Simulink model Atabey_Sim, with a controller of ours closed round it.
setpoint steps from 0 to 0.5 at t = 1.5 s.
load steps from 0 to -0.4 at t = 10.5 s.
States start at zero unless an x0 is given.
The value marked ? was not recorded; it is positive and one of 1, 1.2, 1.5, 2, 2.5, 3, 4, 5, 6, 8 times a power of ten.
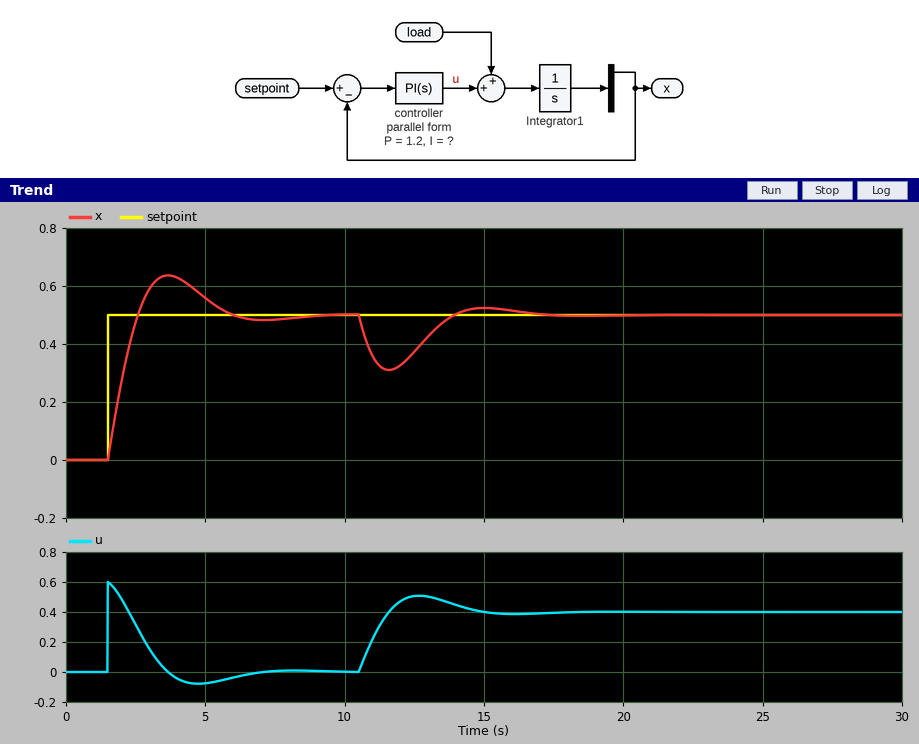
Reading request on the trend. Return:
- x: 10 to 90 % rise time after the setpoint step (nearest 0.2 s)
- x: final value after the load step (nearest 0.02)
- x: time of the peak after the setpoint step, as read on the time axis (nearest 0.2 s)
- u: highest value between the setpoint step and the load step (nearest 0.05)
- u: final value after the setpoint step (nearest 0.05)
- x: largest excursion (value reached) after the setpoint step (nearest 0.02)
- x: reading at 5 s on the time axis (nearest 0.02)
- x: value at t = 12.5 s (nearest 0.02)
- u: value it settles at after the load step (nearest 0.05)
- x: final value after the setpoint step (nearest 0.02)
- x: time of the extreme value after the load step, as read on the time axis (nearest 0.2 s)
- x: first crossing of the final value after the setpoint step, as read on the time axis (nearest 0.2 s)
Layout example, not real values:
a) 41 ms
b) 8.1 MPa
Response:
a) 0.8 s
b) 0.50
c) 3.6 s
d) 0.60
e) 0.00
f) 0.64
g) 0.56
h) 0.38
i) 0.40
j) 0.50
k) 11.6 s
l) 2.6 s
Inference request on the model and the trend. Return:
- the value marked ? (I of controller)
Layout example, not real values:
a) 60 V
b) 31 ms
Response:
a) 1.2
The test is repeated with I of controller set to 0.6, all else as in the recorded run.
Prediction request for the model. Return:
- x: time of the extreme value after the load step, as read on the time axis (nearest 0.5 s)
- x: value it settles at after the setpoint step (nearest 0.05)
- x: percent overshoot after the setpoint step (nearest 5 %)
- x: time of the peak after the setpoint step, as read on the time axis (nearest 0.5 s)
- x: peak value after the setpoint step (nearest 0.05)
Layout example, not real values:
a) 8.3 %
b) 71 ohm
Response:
a) 12.0 s
b) 0.50
c) 20 %
d) 4.5 s
e) 0.60
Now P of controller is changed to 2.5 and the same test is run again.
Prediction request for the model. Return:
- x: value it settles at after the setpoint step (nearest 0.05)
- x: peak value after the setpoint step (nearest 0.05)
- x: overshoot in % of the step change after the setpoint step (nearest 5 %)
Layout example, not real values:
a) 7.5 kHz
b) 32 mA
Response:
a) 0.50
b) 0.55
c) 10 %
